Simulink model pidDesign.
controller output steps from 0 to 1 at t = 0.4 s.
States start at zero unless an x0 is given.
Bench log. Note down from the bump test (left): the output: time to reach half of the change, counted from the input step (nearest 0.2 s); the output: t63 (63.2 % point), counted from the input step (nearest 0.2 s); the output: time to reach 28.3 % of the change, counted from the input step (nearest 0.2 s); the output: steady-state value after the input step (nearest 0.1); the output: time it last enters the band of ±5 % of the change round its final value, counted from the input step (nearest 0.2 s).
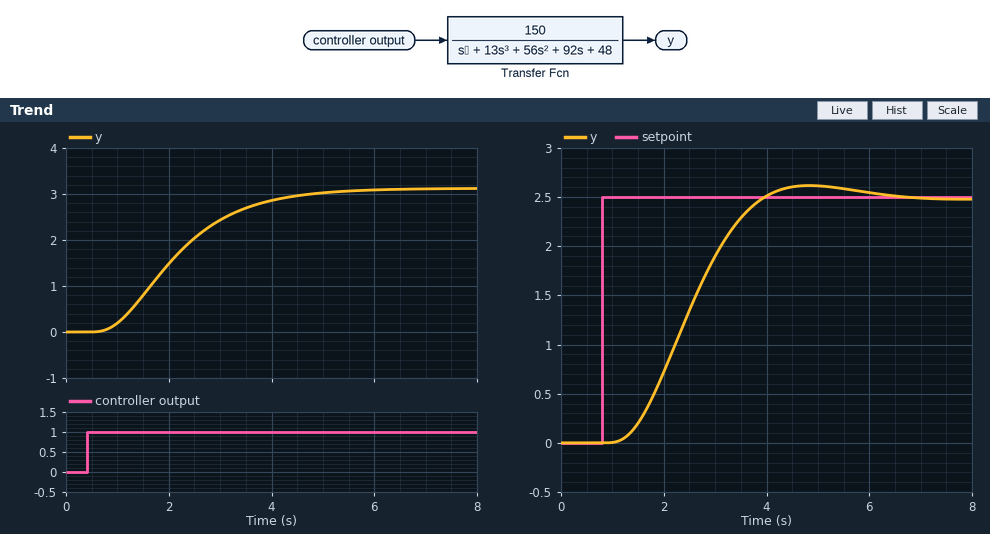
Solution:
1.6 s
2.0 s
1.2 s
3.1
4.2 s
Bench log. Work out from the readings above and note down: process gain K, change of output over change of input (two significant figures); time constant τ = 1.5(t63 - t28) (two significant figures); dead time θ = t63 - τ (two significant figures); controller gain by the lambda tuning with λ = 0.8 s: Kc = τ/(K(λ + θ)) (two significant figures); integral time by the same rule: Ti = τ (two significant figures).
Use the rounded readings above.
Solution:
3.1
1.2 s
0.80 s
0.24
1.2 s
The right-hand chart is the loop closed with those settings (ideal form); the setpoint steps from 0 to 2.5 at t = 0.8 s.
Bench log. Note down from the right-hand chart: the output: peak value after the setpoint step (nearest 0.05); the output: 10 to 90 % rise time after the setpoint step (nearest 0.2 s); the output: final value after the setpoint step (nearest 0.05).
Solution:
2.60
1.8 s
2.50
